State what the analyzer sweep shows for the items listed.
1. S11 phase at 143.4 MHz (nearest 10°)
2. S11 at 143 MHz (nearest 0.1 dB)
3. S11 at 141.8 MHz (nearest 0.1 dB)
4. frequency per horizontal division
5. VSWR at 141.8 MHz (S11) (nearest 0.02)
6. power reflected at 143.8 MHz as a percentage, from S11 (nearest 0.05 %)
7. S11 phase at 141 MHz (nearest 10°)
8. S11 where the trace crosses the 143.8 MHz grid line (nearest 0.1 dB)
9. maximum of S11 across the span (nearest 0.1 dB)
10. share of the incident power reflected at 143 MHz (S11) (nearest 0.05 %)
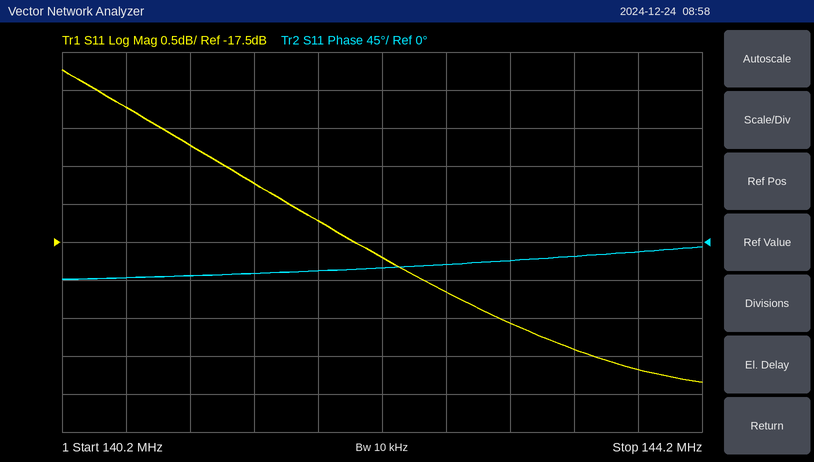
-20°
-18.6 dB
-17.2 dB
400 kHz
1.32
1.20 %
-40°
-19.2 dB
-15.2 dB
1.40 %
